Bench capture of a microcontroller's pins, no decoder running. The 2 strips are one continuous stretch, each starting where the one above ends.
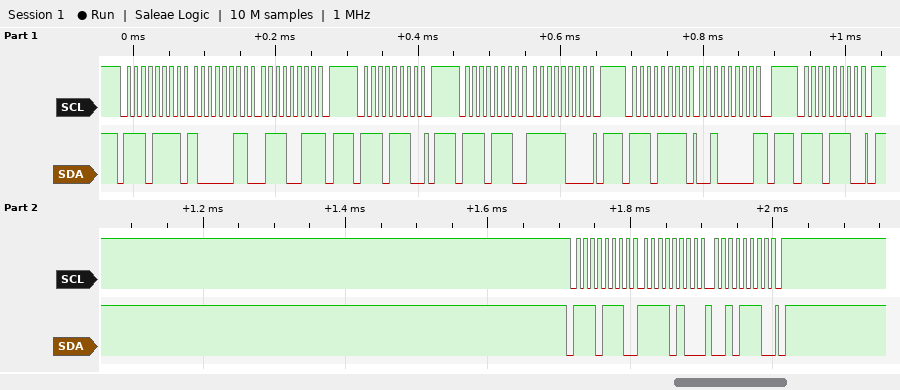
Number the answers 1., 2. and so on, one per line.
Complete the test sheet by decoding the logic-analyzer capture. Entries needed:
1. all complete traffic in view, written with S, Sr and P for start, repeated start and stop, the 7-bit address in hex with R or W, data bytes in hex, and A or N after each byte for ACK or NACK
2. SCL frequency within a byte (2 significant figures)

1. S 77R A 83 A 73 N P S 77W A P S 77W A F8 A P S 77R A 20 N P S 77W A P S 77W A F4 A 2E A P
2. 100 kHz
